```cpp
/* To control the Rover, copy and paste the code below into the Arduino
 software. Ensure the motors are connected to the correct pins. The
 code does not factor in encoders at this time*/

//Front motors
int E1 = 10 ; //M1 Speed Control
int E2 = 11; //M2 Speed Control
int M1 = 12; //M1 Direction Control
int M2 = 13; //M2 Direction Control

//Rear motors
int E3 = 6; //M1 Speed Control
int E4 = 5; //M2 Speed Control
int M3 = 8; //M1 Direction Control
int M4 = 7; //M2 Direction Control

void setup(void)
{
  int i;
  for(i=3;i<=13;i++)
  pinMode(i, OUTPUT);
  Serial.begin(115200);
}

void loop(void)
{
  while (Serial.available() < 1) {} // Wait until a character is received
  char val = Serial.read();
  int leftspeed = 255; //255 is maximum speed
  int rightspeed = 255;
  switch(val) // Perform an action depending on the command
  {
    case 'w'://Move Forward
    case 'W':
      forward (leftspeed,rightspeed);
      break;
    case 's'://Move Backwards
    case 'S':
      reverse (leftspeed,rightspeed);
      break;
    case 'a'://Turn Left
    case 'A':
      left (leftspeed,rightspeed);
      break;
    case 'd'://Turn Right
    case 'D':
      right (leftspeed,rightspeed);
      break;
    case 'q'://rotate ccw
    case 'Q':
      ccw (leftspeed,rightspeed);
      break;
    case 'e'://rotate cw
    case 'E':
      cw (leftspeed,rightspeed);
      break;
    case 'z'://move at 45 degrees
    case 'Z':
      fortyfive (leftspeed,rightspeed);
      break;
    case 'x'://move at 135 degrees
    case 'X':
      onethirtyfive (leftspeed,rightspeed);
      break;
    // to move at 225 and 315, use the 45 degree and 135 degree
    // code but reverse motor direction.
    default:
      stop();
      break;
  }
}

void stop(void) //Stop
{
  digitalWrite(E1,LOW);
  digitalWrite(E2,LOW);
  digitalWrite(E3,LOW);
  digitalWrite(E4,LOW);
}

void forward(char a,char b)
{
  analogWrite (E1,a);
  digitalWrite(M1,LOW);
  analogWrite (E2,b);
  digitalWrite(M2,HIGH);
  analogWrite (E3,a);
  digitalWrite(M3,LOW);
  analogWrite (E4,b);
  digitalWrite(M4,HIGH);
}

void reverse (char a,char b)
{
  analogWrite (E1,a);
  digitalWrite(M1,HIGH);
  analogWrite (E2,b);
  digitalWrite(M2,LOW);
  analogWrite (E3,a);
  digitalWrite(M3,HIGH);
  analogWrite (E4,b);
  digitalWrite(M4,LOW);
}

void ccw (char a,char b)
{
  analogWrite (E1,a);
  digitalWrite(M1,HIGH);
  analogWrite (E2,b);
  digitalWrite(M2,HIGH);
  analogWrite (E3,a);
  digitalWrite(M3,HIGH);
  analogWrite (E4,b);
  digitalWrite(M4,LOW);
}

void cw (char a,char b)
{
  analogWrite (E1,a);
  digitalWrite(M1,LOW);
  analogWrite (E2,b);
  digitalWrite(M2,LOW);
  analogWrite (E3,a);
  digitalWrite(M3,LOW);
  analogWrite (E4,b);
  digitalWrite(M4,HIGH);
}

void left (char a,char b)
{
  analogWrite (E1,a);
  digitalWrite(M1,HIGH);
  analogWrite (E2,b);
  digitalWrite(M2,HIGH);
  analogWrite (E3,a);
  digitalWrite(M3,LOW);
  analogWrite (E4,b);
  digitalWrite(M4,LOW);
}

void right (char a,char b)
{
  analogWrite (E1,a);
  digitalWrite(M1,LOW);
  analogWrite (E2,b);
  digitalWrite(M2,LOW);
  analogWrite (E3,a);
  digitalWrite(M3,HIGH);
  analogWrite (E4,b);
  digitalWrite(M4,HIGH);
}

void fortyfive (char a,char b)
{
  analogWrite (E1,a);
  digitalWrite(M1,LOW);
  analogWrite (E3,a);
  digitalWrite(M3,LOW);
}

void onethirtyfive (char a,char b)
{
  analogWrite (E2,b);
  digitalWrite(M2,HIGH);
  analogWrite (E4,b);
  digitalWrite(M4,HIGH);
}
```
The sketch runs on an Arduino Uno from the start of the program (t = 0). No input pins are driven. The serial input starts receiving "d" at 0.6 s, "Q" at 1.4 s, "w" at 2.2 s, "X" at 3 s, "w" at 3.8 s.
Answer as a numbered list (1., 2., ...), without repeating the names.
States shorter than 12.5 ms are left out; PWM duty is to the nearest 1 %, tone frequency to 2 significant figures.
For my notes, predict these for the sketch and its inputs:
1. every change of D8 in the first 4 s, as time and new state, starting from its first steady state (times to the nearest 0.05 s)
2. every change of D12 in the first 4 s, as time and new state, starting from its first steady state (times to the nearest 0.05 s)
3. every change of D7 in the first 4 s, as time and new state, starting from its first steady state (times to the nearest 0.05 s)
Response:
1. 0 s low; 0.6 s high; 2.2 s low
2. 0 s low; 1.4 s high; 2.2 s low
3. 0 s low; 0.6 s high; 1.4 s low; 2.2 s high
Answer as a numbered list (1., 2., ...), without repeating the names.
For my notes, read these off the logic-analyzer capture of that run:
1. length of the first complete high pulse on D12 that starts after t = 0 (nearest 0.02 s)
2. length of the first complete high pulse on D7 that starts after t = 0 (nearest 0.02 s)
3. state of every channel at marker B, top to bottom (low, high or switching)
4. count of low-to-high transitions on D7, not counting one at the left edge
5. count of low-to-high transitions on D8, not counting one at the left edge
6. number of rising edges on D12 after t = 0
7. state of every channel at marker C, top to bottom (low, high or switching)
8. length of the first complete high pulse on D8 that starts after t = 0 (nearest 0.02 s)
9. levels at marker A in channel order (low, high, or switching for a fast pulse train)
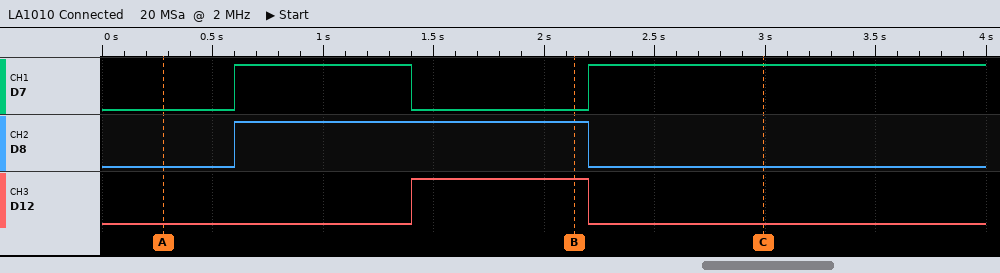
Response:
1. 0.80 s
2. 0.80 s
3. D7 low, D8 high, D12 high
4. 2
5. 1
6. 1
7. D7 high, D8 low, D12 low
8. 1.60 s
9. D7 low, D8 low, D12 low
